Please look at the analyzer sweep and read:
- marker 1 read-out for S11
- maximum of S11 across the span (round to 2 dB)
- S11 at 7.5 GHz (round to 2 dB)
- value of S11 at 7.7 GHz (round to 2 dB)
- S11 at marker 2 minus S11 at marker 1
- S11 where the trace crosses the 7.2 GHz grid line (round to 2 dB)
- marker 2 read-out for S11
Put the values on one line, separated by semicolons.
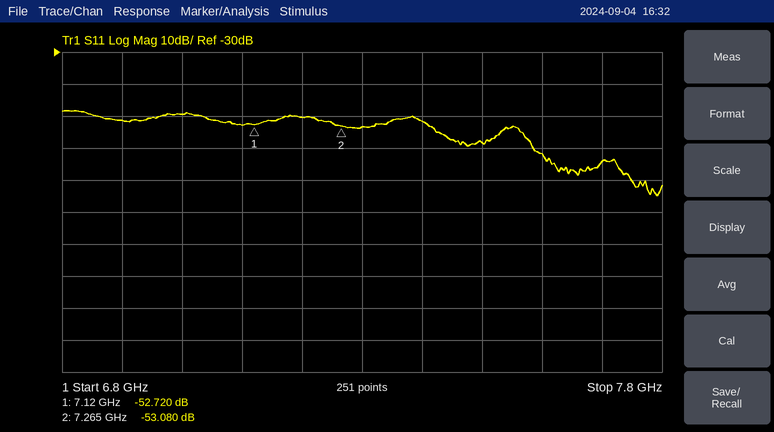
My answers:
-52.720 dB; -48 dB; -58 dB; -64 dB; -0.360 dB; -50 dB; -53.080 dB
